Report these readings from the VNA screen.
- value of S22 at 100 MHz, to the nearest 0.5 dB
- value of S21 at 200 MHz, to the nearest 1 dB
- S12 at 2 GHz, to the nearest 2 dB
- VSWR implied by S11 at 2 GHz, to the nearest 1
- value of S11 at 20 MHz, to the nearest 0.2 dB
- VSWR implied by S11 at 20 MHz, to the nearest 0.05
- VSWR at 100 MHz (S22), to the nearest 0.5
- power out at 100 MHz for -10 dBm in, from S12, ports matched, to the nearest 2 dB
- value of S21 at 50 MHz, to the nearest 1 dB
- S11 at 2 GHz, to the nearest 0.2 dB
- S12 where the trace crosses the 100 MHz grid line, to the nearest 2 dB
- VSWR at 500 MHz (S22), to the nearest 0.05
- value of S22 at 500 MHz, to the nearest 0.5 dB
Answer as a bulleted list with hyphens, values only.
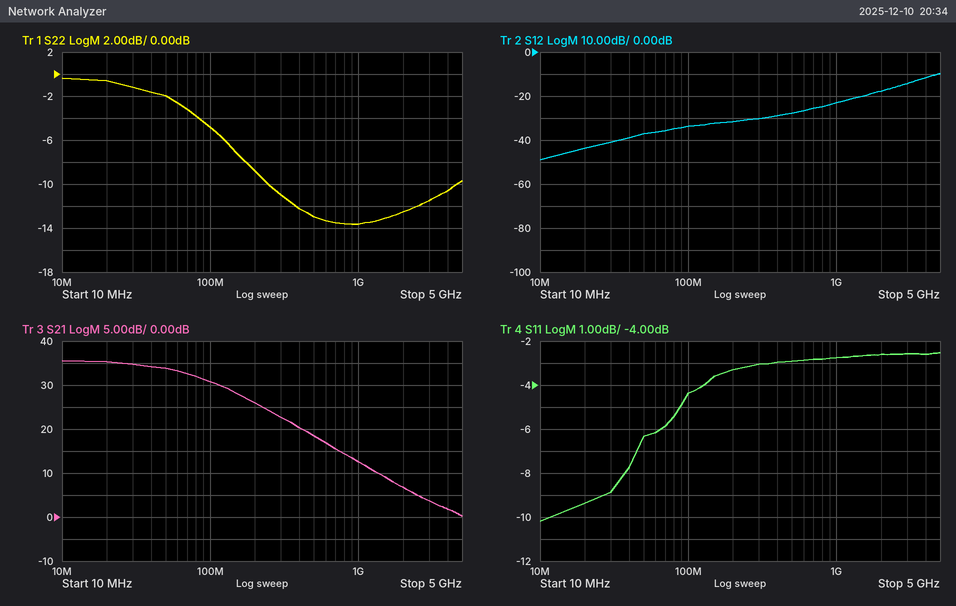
- -5.0 dB
- 26 dB
- -18 dB
- 7
- -9.4 dB
- 2.05
- 3.5
- -44 dBm
- 34 dB
- -2.6 dB
- -34 dB
- 1.60
- -13.0 dB
